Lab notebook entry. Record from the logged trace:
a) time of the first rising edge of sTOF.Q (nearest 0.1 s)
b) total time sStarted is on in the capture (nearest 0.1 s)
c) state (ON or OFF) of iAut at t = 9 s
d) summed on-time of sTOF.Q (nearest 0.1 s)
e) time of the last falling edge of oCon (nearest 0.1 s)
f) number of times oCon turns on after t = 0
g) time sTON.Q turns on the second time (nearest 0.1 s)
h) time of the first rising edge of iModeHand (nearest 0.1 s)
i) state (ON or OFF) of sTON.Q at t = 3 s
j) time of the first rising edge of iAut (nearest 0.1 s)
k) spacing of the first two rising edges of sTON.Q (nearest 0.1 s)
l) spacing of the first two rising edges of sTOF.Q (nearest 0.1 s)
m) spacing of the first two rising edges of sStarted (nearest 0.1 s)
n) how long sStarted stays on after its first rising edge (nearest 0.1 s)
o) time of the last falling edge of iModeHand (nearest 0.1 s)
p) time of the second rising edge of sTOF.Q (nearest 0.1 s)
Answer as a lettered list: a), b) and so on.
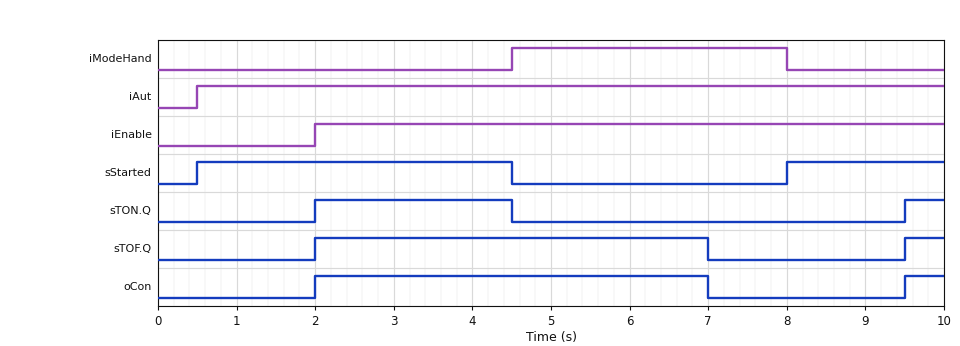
a) 2.0 s
b) 6.0 s
c) ON
d) 5.5 s
e) 7.0 s
f) 2
g) 9.5 s
h) 4.5 s
i) ON
j) 0.5 s
k) 7.5 s
l) 7.5 s
m) 7.5 s
n) 4.0 s
o) 8.0 s
p) 9.5 s
